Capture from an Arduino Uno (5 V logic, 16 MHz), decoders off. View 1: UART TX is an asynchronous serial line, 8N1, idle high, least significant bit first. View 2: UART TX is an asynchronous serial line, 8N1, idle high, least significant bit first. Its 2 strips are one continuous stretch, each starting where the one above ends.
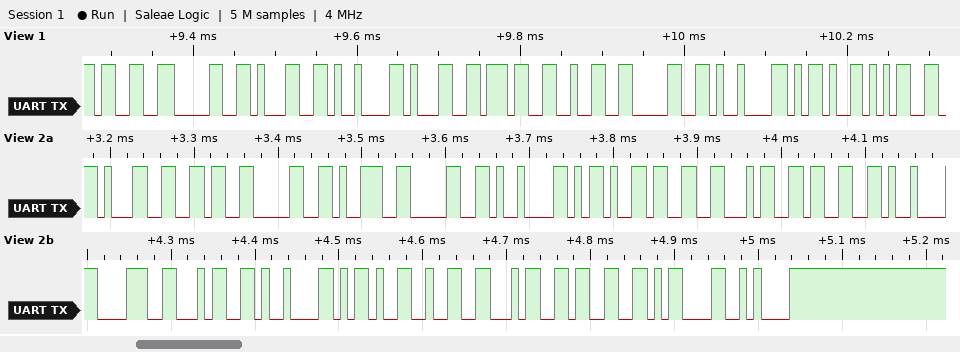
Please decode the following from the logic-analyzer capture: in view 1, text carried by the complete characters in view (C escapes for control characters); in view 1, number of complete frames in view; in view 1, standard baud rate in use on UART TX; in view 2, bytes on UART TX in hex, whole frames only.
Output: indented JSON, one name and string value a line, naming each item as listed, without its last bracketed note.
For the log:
{
  "in view 1, text carried by the complete characters in view": "\"301\\t1720\\t-5\"",
  "in view 1, number of complete frames in view": "11",
  "in view 1, standard baud rate in use on UART TX": "115200 baud",
  "in view 2, bytes on UART TX in hex, whole frames only": "0x31 0x36 0x30 0x39 0x30 0x09 0x2D 0x33 0x34 0x33 0x09 0x38 0x34 0x09 0x2D 0x32 0x34 0x33 0x0D 0x0A"
}
